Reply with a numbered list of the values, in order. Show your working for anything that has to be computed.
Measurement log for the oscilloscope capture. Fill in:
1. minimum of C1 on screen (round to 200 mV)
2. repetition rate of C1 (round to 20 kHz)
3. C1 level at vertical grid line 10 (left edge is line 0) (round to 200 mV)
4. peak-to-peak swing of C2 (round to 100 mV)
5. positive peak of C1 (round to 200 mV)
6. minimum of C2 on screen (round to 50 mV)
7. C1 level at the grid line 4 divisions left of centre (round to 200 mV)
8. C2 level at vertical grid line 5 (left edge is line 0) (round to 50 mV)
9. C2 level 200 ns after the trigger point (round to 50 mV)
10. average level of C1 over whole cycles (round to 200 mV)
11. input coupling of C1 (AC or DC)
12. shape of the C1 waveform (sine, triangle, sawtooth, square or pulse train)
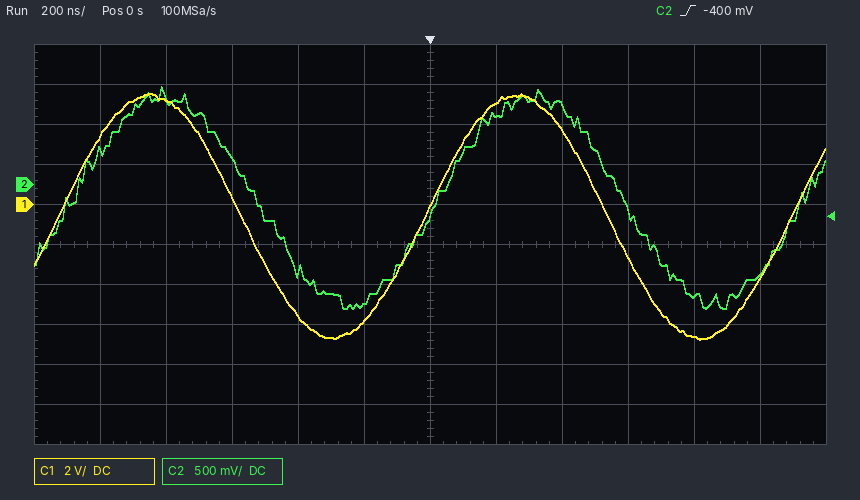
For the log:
1. -6.8 V
2. 900 kHz
3. -6.6 V
4. 2.80 V
5. 5.6 V
6. -1.55 V
7. 5.2 V
8. -1.50 V
9. 850 mV
10. (5.6 V + (-6.8 V)) / 2 ≈ -600 mV
11. DC
12. sine
